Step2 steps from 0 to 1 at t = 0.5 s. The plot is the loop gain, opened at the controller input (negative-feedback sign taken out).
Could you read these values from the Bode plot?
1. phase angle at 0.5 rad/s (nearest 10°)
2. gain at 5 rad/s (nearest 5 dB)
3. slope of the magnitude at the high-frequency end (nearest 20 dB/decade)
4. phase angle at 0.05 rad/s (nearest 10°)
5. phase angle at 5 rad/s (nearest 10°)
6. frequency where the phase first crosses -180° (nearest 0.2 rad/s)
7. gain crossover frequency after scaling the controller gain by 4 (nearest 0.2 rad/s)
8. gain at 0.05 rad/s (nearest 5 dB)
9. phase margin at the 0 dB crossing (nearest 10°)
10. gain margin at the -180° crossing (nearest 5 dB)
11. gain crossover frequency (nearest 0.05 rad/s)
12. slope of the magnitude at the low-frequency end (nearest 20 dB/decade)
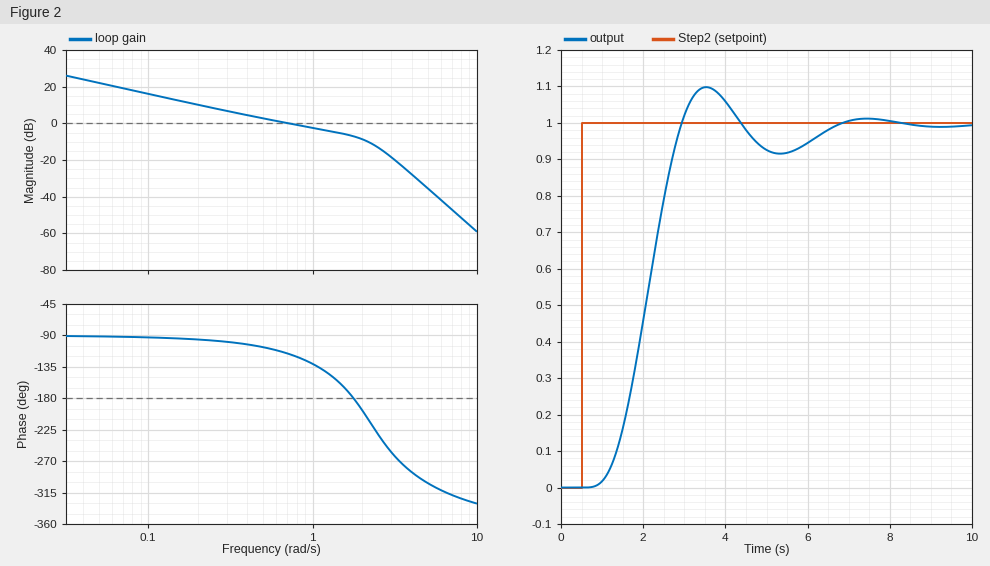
-110°
-35 dB
-80 dB/decade
-90°
-300°
1.8 rad/s
2.4 rad/s
20 dB
60°
5 dB
0.70 rad/s
-20 dB/decade
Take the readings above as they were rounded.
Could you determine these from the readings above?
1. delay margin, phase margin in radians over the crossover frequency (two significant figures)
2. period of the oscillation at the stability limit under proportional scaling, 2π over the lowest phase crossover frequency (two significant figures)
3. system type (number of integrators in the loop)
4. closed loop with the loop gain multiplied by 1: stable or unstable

1.5 s
3.5 s
1
stable
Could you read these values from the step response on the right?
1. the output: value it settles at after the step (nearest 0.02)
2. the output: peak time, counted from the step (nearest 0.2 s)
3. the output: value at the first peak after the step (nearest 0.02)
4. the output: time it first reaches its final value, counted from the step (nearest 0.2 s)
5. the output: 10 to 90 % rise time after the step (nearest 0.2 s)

1.00
3.0 s
1.10
2.4 s
1.4 s
